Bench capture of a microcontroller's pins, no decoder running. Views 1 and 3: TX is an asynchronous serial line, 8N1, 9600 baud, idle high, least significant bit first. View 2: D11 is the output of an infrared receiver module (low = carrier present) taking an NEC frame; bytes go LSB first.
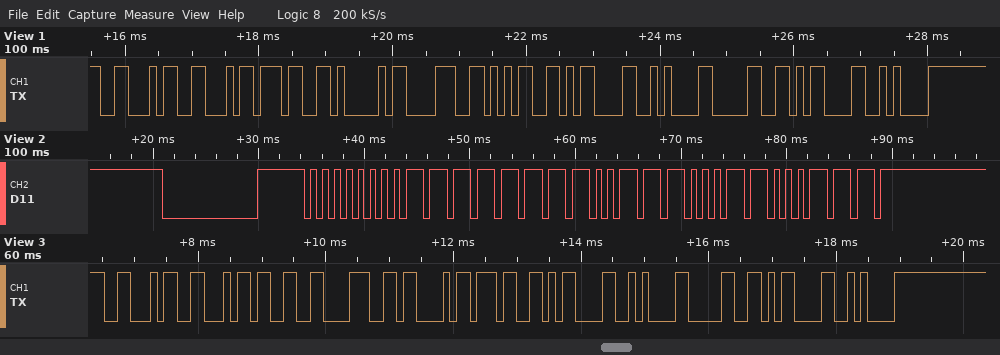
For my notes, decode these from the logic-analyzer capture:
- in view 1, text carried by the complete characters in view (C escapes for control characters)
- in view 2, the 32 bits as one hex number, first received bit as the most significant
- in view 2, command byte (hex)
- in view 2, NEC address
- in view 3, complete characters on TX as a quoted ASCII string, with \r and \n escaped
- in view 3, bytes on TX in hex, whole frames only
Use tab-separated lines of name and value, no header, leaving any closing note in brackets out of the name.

in view 1, text carried by the complete characters in view	"FF7A85\r\n0\r\n"
in view 2, the 32 bits as one hex number, first received bit as the most significant	0x00FF38C7
in view 2, command byte	0x1C
in view 2, NEC address	0x00
in view 3, complete characters on TX as a quoted ASCII string, with \r and \n escaped	"FF38C7\r\n0\r\n"
in view 3, bytes on TX in hex, whole frames only	46 46 33 38 43 37 0D 0A 30 0D 0A
